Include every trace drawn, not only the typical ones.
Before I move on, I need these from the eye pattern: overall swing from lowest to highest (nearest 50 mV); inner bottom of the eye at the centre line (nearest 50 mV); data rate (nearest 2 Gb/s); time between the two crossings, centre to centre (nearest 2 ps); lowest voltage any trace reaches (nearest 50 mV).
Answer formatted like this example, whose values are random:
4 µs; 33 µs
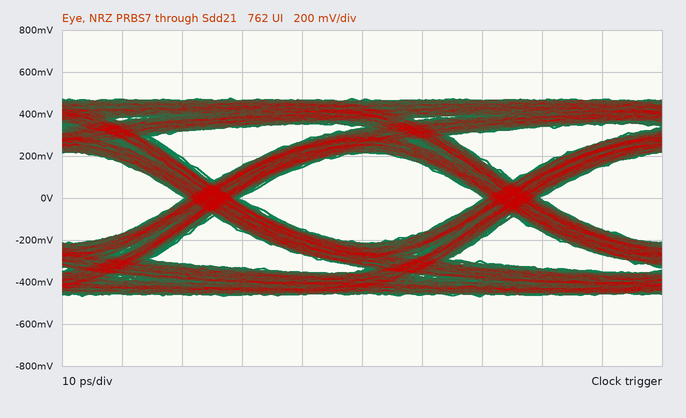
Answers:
950 mV; -200 mV; 20 Gb/s; 50 ps; -450 mV
